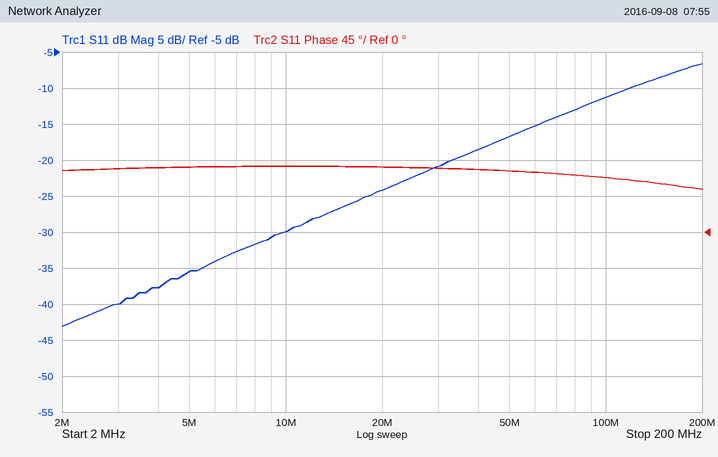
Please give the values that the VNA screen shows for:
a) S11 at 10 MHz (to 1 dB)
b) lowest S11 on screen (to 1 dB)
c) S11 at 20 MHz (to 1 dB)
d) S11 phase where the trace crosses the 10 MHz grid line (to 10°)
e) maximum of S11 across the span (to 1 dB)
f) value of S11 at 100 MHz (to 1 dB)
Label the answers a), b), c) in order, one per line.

a) -30 dB
b) -43 dB
c) -24 dB
d) 80°
e) -7 dB
f) -11 dB
